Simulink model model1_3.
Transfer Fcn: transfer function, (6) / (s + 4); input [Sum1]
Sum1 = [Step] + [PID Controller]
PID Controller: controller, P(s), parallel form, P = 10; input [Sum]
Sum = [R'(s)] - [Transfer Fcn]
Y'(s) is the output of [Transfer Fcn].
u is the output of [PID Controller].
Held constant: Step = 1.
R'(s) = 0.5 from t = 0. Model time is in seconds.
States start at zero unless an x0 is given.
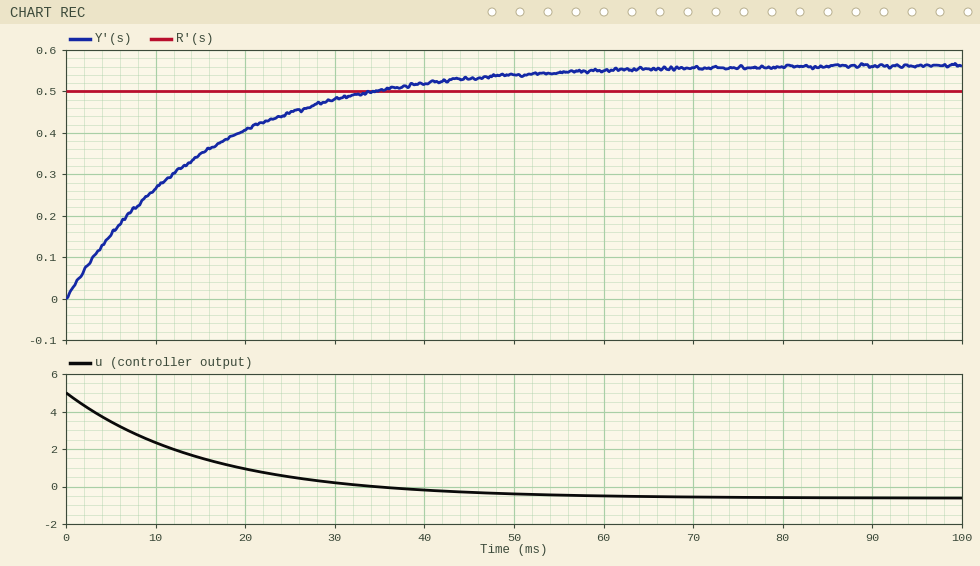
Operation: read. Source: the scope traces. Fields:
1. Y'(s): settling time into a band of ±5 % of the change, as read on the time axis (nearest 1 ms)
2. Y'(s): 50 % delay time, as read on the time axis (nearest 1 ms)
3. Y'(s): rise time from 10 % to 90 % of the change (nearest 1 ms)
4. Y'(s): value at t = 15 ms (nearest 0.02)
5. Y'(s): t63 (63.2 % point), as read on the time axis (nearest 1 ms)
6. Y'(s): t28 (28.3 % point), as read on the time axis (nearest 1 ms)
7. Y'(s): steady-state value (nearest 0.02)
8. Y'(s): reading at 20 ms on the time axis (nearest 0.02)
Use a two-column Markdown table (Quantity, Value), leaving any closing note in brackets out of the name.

| Quantity | Value |
|---|---|
| Y'(s): settling time into a band of ±5 % of the change, as read on the time axis | 47 ms |
| Y'(s): 50 % delay time, as read on the time axis | 11 ms |
| Y'(s): rise time from 10 % to 90 % of the change | 34 ms |
| Y'(s): value at t = 15 ms | 0.34 |
| Y'(s): t63 (63.2 % point), as read on the time axis | 16 ms |
| Y'(s): t28 (28.3 % point), as read on the time axis | 5 ms |
| Y'(s): steady-state value | 0.56 |
| Y'(s): reading at 20 ms on the time axis | 0.40 |
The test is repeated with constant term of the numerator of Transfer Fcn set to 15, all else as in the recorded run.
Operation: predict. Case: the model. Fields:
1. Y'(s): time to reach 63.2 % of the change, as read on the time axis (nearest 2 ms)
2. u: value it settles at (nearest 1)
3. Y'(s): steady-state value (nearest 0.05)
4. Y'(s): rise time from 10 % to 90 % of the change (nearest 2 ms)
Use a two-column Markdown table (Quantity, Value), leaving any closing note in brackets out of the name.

| Quantity | Value |
|---|---|
| Y'(s): time to reach 63.2 % of the change, as read on the time axis | 6 ms |
| u: value it settles at | -1 |
| Y'(s): steady-state value | 0.60 |
| Y'(s): rise time from 10 % to 90 % of the change | 14 ms |
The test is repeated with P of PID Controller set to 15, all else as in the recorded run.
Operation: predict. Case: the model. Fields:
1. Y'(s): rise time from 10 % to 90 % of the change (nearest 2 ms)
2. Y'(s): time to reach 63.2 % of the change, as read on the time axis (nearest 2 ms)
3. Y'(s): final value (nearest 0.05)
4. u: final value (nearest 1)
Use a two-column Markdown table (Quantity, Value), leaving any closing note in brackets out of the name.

| Quantity | Value |
|---|---|
| Y'(s): rise time from 10 % to 90 % of the change | 24 ms |
| Y'(s): time to reach 63.2 % of the change, as read on the time axis | 10 ms |
| Y'(s): final value | 0.55 |
| u: final value | -1 |
